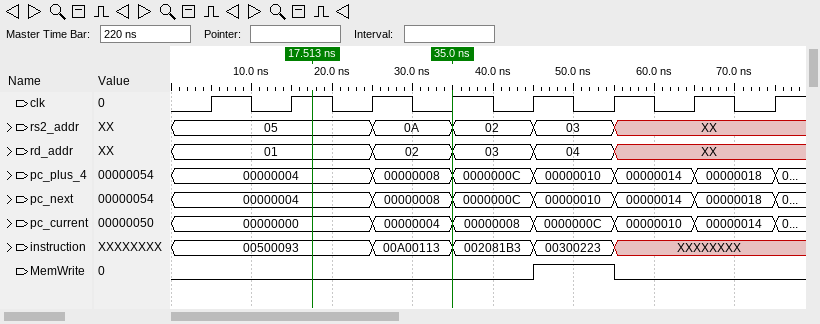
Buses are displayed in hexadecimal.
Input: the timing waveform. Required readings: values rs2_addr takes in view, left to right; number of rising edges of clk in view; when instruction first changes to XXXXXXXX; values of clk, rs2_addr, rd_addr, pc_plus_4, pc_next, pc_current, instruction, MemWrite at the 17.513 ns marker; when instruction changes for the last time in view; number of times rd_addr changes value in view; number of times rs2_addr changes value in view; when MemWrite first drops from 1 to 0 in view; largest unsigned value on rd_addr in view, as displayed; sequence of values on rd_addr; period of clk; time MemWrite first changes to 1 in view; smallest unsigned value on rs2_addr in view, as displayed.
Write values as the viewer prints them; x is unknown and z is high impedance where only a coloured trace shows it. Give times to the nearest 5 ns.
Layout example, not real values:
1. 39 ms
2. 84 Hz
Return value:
1. 05, 0A, 02, 03, XX
2. 8
3. 55 ns
4. clk=1, rs2_addr=05, rd_addr=01, pc_plus_4=00000004, pc_next=00000004, pc_current=00000000, instruction=00500093, MemWrite=0
5. 55 ns
6. 4
7. 4
8. 55 ns
9. 04
10. 01, 02, 03, 04, XX
11. 10 ns
12. 45 ns
13. 02
